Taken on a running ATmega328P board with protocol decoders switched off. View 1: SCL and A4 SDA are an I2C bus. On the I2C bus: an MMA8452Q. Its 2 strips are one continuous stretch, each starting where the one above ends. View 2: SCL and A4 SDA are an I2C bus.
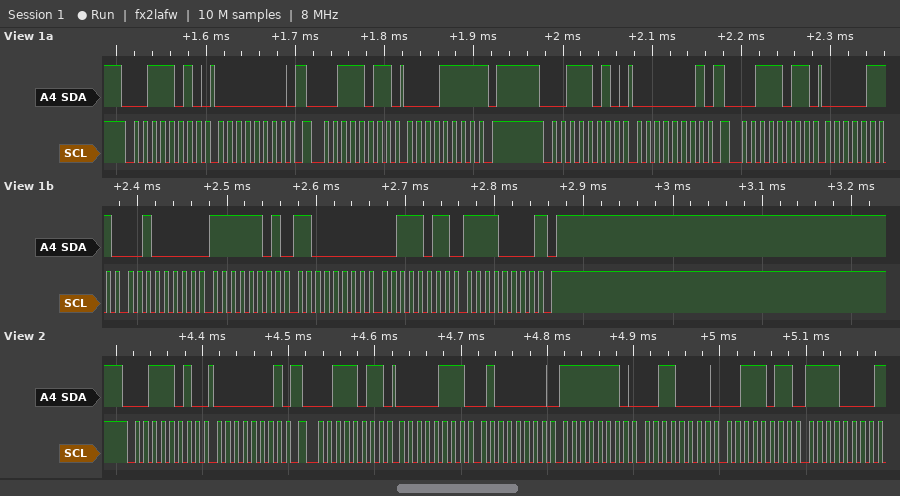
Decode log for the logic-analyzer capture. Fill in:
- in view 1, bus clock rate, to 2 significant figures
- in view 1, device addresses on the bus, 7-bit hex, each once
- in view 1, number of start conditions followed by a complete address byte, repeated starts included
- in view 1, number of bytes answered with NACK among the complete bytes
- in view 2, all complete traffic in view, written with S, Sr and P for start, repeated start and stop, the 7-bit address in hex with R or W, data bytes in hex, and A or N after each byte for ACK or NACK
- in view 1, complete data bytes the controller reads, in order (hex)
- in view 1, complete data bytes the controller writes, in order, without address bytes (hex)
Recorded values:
100 kHz
0x1D
4
2
S 1DW A 01 A Sr 1DR A 07 A 40 A FE A 30 A 3B A F0 N
0F 07 20 FD C0 3B F0
00 01
